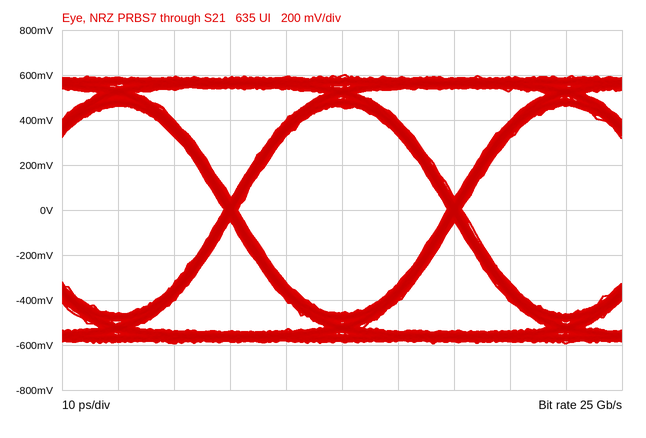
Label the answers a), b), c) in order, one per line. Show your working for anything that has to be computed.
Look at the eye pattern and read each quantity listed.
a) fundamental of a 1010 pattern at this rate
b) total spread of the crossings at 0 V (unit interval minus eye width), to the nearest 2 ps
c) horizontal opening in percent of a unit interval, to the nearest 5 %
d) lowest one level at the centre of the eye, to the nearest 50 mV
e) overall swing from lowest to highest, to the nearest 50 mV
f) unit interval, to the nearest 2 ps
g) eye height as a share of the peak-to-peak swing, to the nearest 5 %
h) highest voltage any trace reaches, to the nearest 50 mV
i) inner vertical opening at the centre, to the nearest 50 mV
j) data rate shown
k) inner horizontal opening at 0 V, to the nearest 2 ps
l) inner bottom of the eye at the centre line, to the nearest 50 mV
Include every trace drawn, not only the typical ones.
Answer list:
a) 12.5 GHz
b) 2 ps
c) 38 ps / 40 ps ≈ 95 %
d) 450 mV
e) 1.20 V
f) 40 ps
g) 900 mV / 1.20 V ≈ 75 %
h) 600 mV
i) 900 mV
j) 25 Gb/s
k) 38 ps
l) -450 mV
